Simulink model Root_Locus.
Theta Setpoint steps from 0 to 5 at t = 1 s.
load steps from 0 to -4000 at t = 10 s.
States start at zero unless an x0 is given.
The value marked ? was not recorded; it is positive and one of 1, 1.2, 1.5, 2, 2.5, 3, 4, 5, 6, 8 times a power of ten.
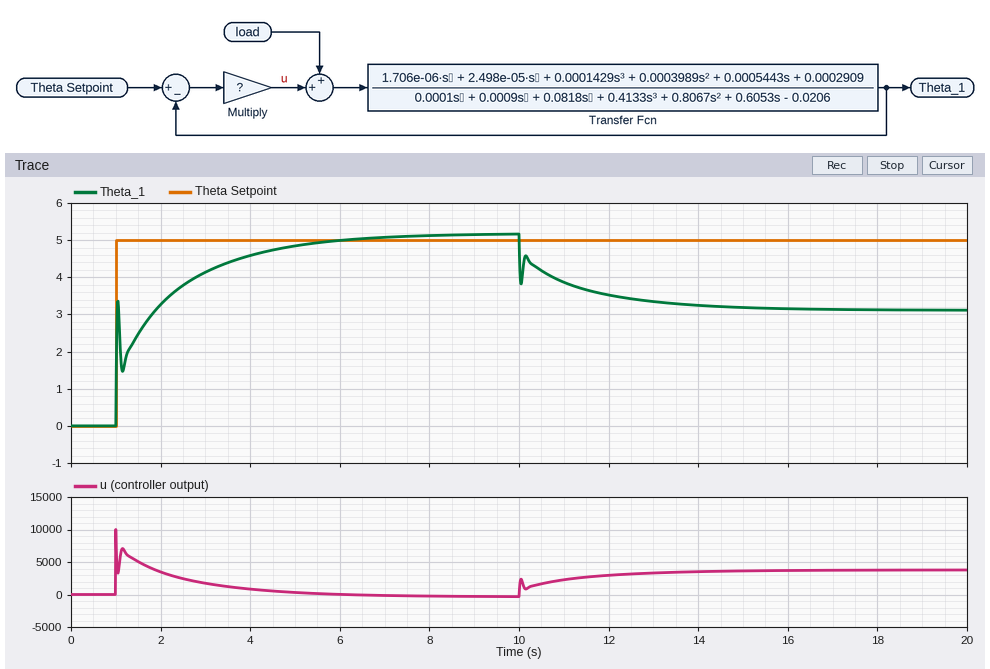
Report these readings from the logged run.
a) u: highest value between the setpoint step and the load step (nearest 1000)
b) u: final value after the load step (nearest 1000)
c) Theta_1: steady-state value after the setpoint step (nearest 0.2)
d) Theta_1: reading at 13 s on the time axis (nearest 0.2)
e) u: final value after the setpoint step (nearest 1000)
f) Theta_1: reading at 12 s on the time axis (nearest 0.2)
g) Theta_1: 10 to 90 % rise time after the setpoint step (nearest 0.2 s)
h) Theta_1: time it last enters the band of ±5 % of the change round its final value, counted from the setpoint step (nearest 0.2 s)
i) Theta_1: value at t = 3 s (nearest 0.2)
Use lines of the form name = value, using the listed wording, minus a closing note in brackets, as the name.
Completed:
u: highest value between the setpoint step and the load step = 10000
u: final value after the load step = 4000
Theta_1: steady-state value after the setpoint step = 5.2
Theta_1: reading at 13 s on the time axis = 3.4
u: final value after the setpoint step = 0
Theta_1: reading at 12 s on the time axis = 3.6
Theta_1: 10 to 90 % rise time after the setpoint step = 3.2 s
Theta_1: time it last enters the band of ±5 % of the change round its final value, counted from the setpoint step = 4.4 s
Theta_1: value at t = 3 s = 4.2
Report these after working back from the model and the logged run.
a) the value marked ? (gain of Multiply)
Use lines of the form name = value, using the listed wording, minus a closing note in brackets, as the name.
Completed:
the value marked ? = 2000
